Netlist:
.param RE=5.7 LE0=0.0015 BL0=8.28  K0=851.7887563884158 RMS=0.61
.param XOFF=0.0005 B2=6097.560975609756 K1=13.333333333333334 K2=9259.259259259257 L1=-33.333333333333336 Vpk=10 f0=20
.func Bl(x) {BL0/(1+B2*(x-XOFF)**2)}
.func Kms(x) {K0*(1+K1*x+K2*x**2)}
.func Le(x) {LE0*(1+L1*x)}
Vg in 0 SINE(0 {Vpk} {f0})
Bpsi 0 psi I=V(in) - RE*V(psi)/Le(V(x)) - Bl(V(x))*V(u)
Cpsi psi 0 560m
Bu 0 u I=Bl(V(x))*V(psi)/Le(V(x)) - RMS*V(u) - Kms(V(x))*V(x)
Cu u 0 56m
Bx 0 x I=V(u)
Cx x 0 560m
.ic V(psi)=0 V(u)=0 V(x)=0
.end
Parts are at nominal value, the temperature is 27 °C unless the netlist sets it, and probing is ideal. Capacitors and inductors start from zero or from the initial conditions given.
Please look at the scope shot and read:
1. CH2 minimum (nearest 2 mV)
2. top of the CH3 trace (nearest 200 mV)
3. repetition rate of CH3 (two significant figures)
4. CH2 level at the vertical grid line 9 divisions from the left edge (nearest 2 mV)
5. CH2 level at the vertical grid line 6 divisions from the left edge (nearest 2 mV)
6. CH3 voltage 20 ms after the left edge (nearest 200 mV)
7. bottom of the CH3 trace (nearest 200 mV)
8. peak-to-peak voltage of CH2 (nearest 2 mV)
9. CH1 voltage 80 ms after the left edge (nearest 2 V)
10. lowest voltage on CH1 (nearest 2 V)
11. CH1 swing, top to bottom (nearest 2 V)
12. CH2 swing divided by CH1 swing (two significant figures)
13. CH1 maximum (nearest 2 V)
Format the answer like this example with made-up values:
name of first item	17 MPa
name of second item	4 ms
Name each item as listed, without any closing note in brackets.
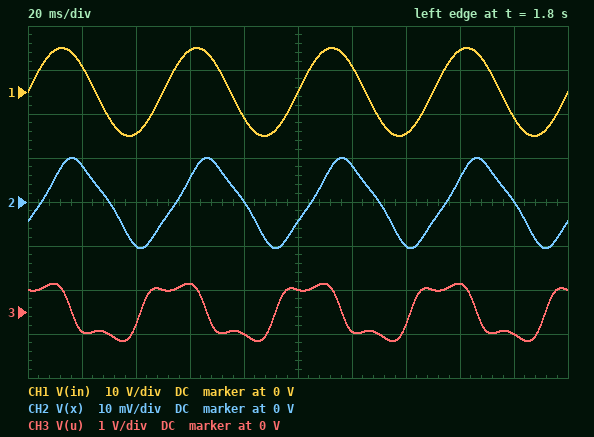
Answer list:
CH2 minimum	-10 mV
top of the CH3 trace	600 mV
repetition rate of CH3	20 Hz
CH2 level at the vertical grid line 9 divisions from the left edge	0 V
CH2 level at the vertical grid line 6 divisions from the left edge	8 mV
CH3 voltage 20 ms after the left edge	-400 mV
bottom of the CH3 trace	-600 mV
peak-to-peak voltage of CH2	20 mV
CH1 voltage 80 ms after the left edge	-6 V
lowest voltage on CH1	-10 V
CH1 swing, top to bottom	20 V
CH2 swing divided by CH1 swing	0.0010
CH1 maximum	10 V
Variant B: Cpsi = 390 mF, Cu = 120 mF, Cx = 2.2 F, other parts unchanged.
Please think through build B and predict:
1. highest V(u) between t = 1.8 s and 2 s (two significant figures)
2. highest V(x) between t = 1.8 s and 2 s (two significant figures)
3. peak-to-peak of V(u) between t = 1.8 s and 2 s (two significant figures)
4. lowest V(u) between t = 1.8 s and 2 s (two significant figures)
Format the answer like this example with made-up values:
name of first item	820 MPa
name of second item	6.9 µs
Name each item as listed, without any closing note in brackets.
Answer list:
highest V(u) between t = 1.8 s and 2 s	840 mV
highest V(x) between t = 1.8 s and 2 s	2.8 mV
peak-to-peak of V(u) between t = 1.8 s and 2 s	1.7 V
lowest V(u) between t = 1.8 s and 2 s	-830 mV
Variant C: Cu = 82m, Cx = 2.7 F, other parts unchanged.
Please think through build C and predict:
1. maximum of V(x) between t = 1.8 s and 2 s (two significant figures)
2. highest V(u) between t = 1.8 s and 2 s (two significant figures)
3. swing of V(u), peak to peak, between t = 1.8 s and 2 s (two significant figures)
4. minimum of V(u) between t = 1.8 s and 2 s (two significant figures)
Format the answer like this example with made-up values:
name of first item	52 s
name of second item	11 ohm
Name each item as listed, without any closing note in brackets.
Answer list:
maximum of V(x) between t = 1.8 s and 2 s	2.8 mV
highest V(u) between t = 1.8 s and 2 s	1.0 V
swing of V(u), peak to peak, between t = 1.8 s and 2 s	2.0 V
minimum of V(u) between t = 1.8 s and 2 s	-980 mV
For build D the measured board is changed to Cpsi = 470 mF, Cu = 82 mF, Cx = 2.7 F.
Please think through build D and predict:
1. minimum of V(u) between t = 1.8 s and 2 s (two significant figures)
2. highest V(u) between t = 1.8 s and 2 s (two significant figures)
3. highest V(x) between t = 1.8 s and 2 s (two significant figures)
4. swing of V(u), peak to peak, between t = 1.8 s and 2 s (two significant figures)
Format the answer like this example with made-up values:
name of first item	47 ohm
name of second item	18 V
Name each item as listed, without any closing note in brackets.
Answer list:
minimum of V(u) between t = 1.8 s and 2 s	-980 mV
highest V(u) between t = 1.8 s and 2 s	1.0 V
highest V(x) between t = 1.8 s and 2 s	2.8 mV
swing of V(u), peak to peak, between t = 1.8 s and 2 s	2.0 V
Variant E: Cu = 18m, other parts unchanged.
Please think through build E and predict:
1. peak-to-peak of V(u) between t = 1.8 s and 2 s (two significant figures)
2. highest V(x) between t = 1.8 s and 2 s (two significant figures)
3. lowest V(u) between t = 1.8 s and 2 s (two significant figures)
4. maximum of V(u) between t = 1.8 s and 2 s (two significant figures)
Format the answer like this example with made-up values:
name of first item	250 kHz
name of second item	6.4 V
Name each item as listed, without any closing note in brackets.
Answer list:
peak-to-peak of V(u) between t = 1.8 s and 2 s	1.4 V
highest V(x) between t = 1.8 s and 2 s	8.5 mV
lowest V(u) between t = 1.8 s and 2 s	-720 mV
maximum of V(u) between t = 1.8 s and 2 s	710 mV
